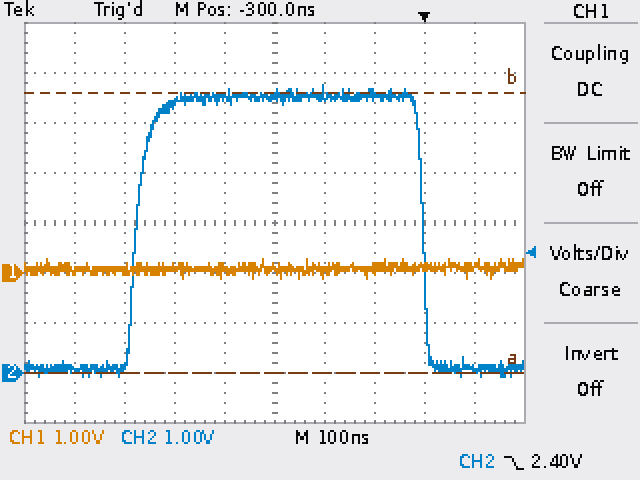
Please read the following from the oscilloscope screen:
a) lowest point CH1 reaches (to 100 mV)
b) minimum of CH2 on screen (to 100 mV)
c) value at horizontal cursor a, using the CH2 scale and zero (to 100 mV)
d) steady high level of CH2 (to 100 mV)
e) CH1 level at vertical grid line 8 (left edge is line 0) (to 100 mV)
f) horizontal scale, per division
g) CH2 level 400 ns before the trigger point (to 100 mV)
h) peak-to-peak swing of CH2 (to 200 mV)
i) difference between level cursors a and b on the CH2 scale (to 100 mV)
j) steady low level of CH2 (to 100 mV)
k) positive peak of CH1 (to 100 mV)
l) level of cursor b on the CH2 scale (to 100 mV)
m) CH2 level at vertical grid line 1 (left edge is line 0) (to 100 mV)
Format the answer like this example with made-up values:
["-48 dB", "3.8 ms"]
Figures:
["-100 mV", "-100 mV", "0.0 V", "5.5 V", "100 mV", "100 ns", "5.5 V", "5.8 V", "5.6 V", "100 mV", "300 mV", "5.6 V", "100 mV"]
